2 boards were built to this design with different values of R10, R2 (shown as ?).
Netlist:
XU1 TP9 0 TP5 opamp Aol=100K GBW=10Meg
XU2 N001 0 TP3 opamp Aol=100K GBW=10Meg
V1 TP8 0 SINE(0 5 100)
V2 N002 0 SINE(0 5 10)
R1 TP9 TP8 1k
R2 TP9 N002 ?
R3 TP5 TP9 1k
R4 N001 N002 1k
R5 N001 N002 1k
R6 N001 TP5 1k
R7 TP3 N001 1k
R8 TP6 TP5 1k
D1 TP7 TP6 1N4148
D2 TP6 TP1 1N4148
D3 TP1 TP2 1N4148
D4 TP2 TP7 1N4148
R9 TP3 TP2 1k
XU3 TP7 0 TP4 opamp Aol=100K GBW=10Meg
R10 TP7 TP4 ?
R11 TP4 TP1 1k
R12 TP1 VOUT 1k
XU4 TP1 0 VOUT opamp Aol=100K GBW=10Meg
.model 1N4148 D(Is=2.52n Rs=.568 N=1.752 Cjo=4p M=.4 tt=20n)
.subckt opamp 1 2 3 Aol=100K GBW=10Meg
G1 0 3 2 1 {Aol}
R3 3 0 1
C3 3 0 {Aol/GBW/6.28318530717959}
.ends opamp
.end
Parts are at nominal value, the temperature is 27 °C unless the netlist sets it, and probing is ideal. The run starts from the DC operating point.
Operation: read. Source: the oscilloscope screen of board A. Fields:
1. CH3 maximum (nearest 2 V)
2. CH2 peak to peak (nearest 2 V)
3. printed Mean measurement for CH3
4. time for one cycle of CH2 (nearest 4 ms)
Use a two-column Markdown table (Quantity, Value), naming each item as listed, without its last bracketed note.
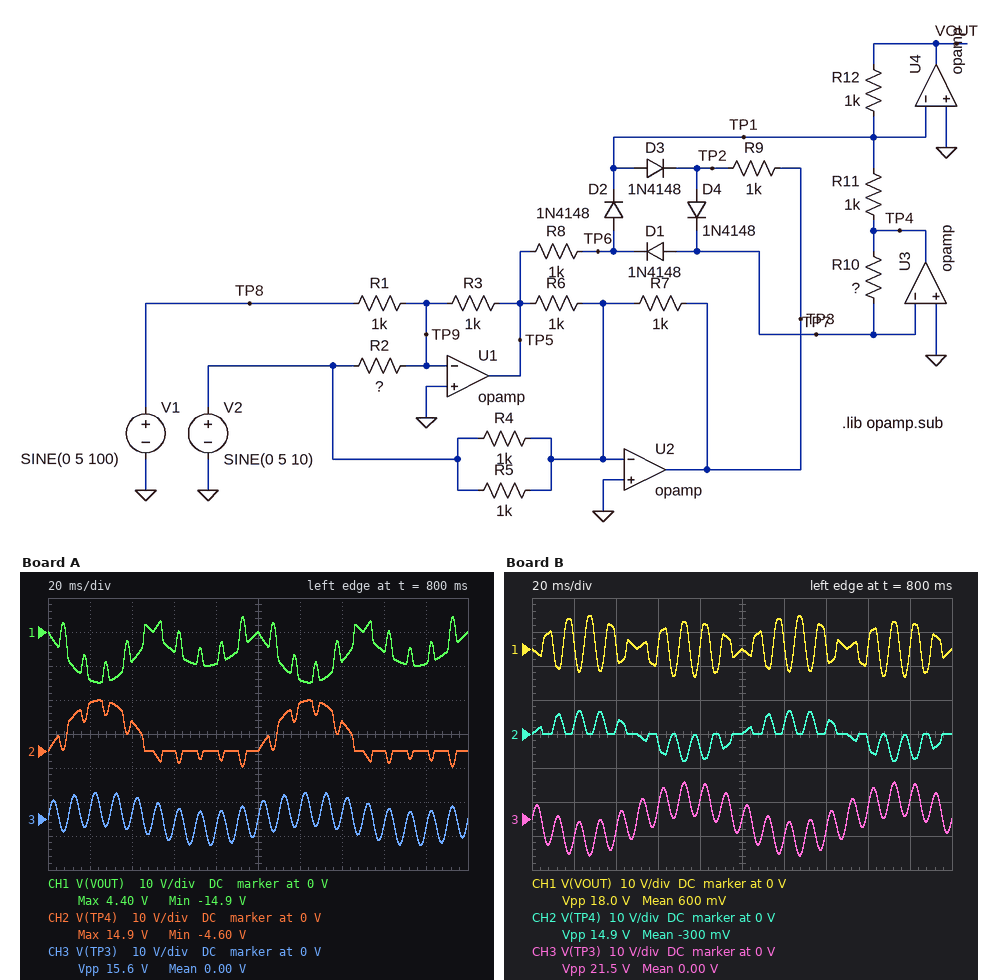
| Quantity | Value |
|---|---|
| CH3 maximum | 8 V |
| CH2 peak to peak | 20 V |
| printed Mean measurement for CH3 | 0.00 V |
| time for one cycle of CH2 | 100 ms |
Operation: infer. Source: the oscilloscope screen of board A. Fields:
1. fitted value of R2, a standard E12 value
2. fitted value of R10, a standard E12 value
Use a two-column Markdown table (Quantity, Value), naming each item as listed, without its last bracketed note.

| Quantity | Value |
|---|---|
| fitted value of R2, a standard E12 value | 390 Ω |
| fitted value of R10, a standard E12 value | 1.5 kΩ |
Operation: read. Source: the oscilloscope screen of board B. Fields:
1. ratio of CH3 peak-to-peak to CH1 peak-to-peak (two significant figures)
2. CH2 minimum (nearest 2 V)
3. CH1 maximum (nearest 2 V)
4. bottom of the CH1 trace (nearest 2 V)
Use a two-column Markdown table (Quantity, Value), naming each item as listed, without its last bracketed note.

| Quantity | Value |
|---|---|
| ratio of CH3 peak-to-peak to CH1 peak-to-peak | 1.2 |
| CH2 minimum | -8 V |
| CH1 maximum | 10 V |
| bottom of the CH1 trace | -8 V |
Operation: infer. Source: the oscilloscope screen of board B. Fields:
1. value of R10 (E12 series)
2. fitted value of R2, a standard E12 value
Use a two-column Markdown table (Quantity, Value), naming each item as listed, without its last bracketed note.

| Quantity | Value |
|---|---|
| value of R10 | 820 Ω |
| fitted value of R2, a standard E12 value | 1.2 kΩ |
